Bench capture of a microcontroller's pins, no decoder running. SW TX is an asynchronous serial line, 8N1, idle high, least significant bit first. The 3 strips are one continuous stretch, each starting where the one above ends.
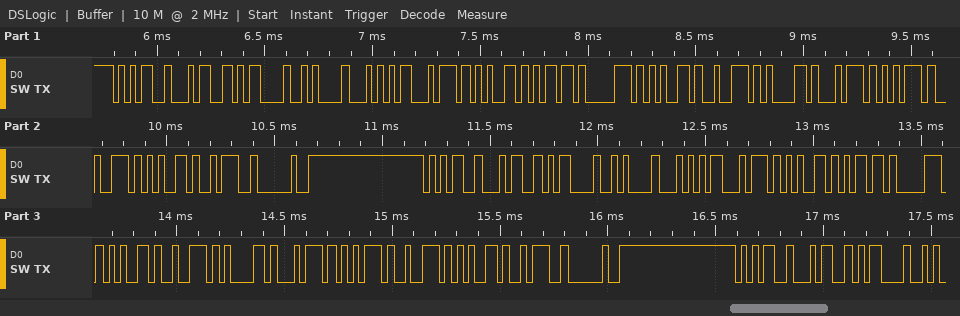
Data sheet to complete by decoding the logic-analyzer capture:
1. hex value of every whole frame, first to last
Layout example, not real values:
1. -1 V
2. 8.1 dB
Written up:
1. 35 34 0D 0A 54 74 65 6D 70 65 72 61 74 75 72 65 3A 20 35 34 0D 0A 54 74 65 6D 70 65 72 61 74 75 72 65 3A 20 35 34 0D
